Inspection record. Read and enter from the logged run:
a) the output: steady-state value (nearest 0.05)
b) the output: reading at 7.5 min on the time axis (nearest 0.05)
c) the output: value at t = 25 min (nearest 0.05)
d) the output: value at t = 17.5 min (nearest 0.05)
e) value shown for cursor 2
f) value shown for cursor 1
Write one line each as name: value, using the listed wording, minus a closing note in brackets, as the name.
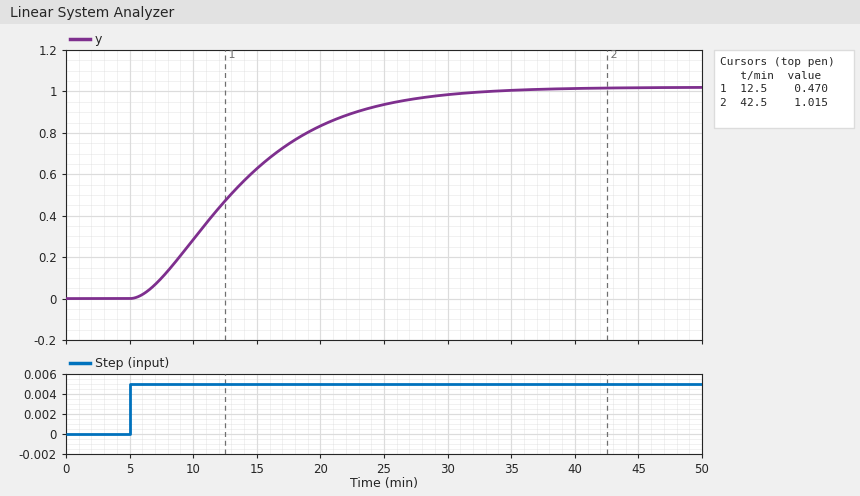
the output: steady-state value: 1.00
the output: reading at 7.5 min on the time axis: 0.10
the output: value at t = 25 min: 0.95
the output: value at t = 17.5 min: 0.75
value shown for cursor 2: 1.015
value shown for cursor 1: 0.470
